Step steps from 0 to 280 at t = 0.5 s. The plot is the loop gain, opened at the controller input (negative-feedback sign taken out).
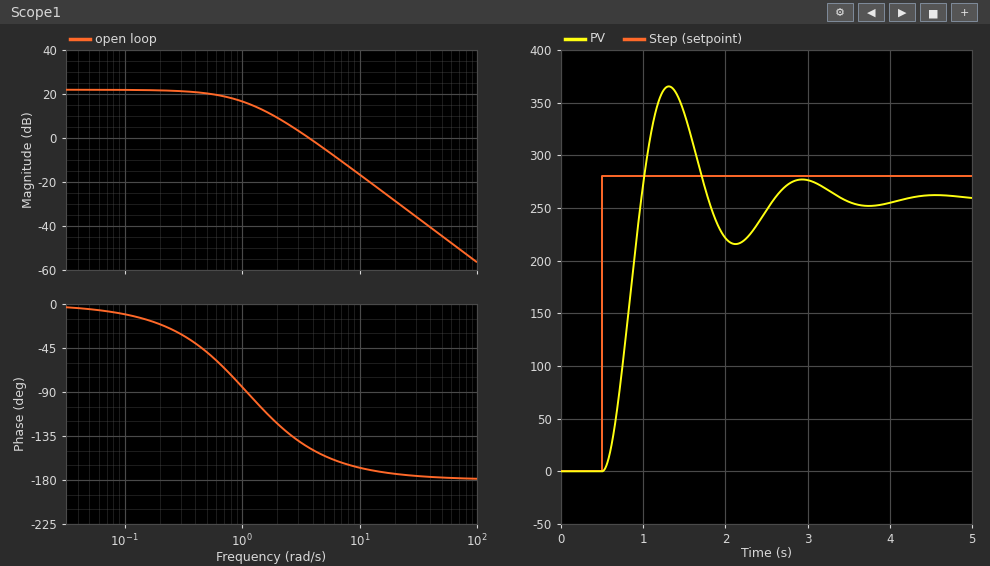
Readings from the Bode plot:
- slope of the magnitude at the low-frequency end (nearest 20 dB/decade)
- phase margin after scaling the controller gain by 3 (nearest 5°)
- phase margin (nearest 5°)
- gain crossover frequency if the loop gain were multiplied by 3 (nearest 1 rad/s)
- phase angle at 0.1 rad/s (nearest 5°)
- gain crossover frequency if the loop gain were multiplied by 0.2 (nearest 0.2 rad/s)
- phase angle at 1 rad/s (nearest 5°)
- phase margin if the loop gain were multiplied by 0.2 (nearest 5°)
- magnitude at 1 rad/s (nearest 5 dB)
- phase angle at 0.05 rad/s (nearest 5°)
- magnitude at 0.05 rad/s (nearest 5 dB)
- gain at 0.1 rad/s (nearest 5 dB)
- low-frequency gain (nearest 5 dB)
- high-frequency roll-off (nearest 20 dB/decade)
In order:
0 dB/decade
20°
35°
7 rad/s
-10°
1.4 rad/s
-85°
80°
15 dB
-5°
20 dB
20 dB
20 dB
-40 dB/decade
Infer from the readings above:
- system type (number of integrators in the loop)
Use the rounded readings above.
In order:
0
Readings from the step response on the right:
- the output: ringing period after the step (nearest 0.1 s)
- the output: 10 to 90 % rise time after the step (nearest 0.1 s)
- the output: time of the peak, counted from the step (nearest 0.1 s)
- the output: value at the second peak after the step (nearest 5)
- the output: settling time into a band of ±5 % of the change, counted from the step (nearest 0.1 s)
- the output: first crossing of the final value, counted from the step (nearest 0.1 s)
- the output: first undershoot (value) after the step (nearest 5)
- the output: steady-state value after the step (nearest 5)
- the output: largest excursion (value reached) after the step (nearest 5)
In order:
1.6 s
0.3 s
0.8 s
275
2.6 s
0.5 s
215
260
365
